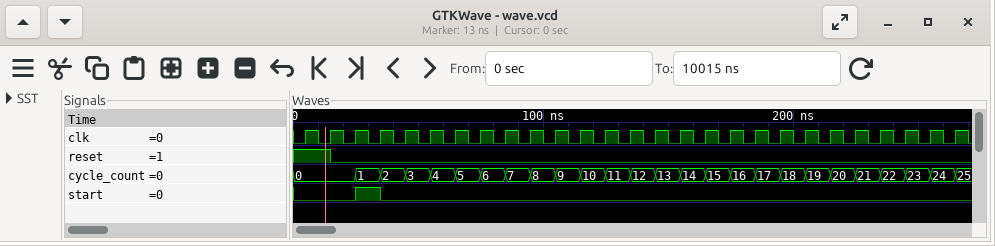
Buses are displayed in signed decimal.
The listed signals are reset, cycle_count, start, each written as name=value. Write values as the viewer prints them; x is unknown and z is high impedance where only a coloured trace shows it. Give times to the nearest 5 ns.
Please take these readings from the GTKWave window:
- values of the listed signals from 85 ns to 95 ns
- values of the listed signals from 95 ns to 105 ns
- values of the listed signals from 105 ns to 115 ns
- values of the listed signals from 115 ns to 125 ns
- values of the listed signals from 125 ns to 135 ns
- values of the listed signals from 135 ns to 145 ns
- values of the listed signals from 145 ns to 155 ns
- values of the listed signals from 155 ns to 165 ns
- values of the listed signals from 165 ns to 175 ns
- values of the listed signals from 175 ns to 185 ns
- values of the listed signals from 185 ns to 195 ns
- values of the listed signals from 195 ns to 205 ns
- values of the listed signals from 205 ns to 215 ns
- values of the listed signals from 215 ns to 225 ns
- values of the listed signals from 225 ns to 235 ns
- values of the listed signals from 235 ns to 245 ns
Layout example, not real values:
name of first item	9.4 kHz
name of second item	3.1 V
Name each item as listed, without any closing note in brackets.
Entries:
values of the listed signals from 85 ns to 95 ns	reset=0, cycle_count=7, start=0
values of the listed signals from 95 ns to 105 ns	reset=0, cycle_count=8, start=0
values of the listed signals from 105 ns to 115 ns	reset=0, cycle_count=9, start=0
values of the listed signals from 115 ns to 125 ns	reset=0, cycle_count=10, start=0
values of the listed signals from 125 ns to 135 ns	reset=0, cycle_count=11, start=0
values of the listed signals from 135 ns to 145 ns	reset=0, cycle_count=12, start=0
values of the listed signals from 145 ns to 155 ns	reset=0, cycle_count=13, start=0
values of the listed signals from 155 ns to 165 ns	reset=0, cycle_count=14, start=0
values of the listed signals from 165 ns to 175 ns	reset=0, cycle_count=15, start=0
values of the listed signals from 175 ns to 185 ns	reset=0, cycle_count=16, start=0
values of the listed signals from 185 ns to 195 ns	reset=0, cycle_count=17, start=0
values of the listed signals from 195 ns to 205 ns	reset=0, cycle_count=18, start=0
values of the listed signals from 205 ns to 215 ns	reset=0, cycle_count=19, start=0
values of the listed signals from 215 ns to 225 ns	reset=0, cycle_count=20, start=0
values of the listed signals from 225 ns to 235 ns	reset=0, cycle_count=21, start=0
values of the listed signals from 235 ns to 245 ns	reset=0, cycle_count=22, start=0
